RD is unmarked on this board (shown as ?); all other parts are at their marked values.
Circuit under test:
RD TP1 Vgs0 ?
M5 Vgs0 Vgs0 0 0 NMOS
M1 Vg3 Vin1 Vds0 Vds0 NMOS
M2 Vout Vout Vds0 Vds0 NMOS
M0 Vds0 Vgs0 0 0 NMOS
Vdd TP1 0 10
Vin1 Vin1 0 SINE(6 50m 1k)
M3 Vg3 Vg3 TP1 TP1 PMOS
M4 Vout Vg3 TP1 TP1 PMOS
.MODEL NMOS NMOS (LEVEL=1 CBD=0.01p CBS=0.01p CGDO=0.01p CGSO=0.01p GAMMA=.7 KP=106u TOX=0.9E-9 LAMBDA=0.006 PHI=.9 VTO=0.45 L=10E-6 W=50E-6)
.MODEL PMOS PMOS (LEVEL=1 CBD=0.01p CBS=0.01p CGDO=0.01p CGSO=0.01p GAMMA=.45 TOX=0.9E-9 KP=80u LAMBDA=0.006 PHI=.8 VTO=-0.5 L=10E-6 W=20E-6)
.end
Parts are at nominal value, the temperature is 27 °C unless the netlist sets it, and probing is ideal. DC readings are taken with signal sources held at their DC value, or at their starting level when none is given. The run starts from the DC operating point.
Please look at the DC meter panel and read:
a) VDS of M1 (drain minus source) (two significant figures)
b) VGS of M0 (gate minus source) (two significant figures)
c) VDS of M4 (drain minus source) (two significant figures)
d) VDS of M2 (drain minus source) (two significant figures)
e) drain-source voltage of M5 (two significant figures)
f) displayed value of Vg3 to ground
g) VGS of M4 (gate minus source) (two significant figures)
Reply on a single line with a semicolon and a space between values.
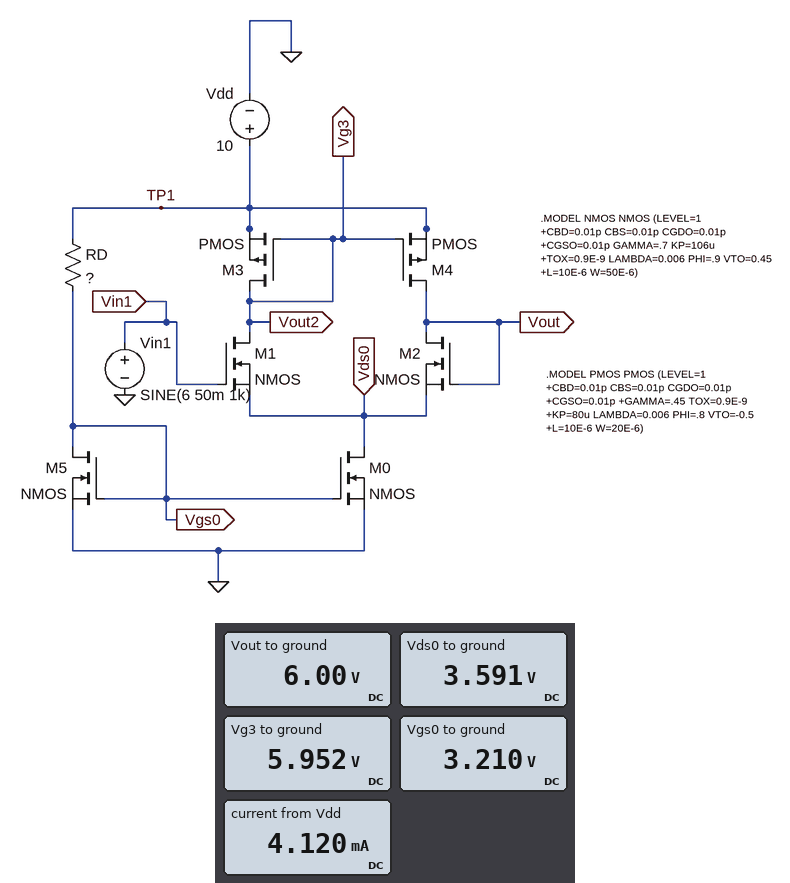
2.4 V; 3.2 V; -4.0 V; 2.4 V; 3.2 V; 5.952 V; -4.0 V
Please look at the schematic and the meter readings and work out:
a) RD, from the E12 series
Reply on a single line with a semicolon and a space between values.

3.3 kΩ
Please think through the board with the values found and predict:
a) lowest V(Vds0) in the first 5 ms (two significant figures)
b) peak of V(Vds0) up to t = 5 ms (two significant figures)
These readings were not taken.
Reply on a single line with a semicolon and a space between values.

3.5 V; 3.6 V
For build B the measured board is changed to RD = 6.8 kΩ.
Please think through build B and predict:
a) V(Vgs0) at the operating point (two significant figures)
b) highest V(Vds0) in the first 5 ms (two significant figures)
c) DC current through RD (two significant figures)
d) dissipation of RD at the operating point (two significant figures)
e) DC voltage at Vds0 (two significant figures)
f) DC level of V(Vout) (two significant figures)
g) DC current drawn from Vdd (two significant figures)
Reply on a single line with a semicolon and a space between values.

2.5 V; 4.2 V; 1.1 mA; 8.3 mW; 4.1 V; 6.0 V; 2.2 mA
